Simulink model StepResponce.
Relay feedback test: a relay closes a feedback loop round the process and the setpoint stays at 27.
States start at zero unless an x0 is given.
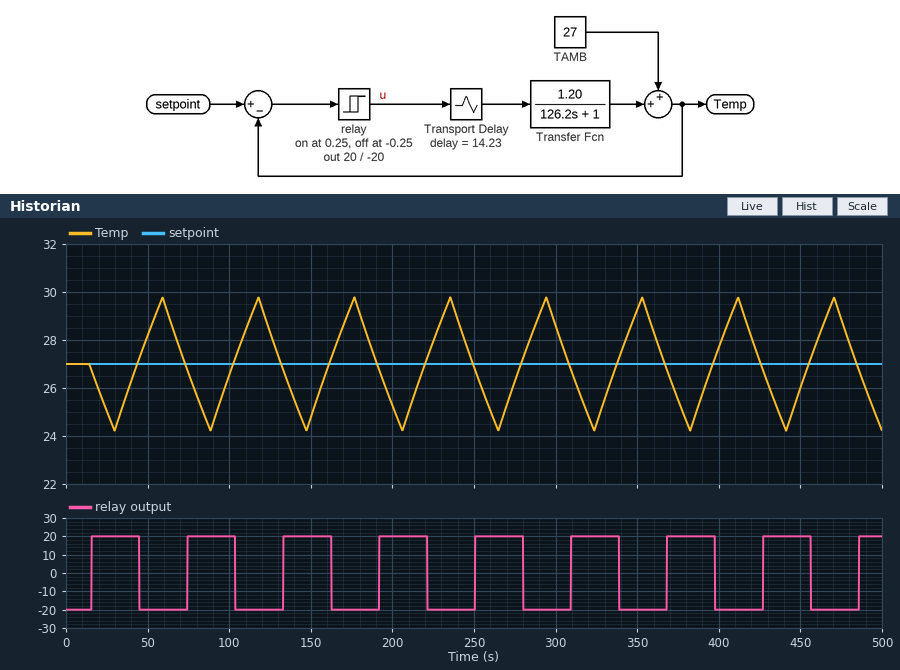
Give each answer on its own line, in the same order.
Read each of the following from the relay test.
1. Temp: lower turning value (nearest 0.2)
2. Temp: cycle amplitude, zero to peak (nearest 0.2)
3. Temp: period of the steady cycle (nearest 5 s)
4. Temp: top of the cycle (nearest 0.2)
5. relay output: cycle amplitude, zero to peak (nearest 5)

24.2
2.8
60 s
29.8
20
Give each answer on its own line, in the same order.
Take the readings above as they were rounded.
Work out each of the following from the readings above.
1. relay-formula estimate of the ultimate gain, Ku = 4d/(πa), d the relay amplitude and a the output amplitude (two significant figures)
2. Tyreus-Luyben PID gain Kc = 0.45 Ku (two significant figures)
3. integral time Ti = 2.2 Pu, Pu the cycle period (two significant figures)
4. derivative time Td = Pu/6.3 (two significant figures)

9.1
4.1
130 s
9.5 s
